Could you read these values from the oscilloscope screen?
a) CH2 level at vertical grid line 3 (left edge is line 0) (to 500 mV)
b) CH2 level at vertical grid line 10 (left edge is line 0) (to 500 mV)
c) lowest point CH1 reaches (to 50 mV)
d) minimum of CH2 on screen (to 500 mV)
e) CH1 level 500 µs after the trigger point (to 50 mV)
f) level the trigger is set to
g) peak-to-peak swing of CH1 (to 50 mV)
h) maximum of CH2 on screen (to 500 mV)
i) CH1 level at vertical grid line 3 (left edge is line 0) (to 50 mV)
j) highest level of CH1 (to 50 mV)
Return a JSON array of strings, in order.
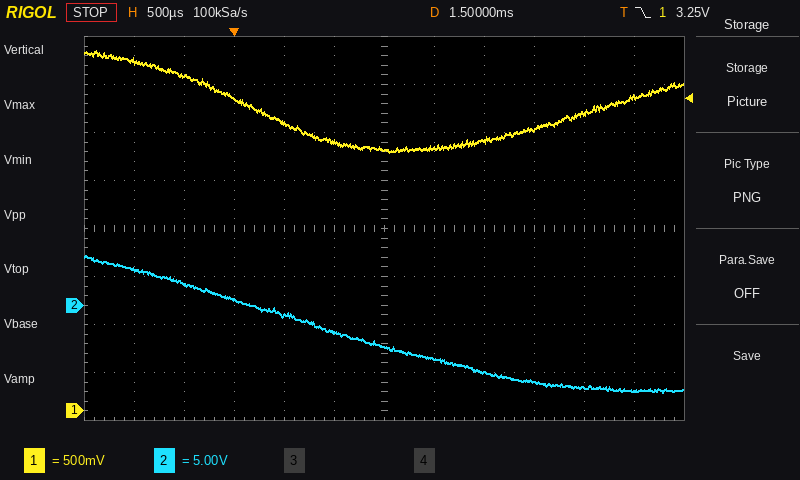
["500 mV", "-8.5 V", "2.70 V", "-9.0 V", "3.00 V", "3.25 V", "1.05 V", "5.0 V", "3.25 V", "3.75 V"]
